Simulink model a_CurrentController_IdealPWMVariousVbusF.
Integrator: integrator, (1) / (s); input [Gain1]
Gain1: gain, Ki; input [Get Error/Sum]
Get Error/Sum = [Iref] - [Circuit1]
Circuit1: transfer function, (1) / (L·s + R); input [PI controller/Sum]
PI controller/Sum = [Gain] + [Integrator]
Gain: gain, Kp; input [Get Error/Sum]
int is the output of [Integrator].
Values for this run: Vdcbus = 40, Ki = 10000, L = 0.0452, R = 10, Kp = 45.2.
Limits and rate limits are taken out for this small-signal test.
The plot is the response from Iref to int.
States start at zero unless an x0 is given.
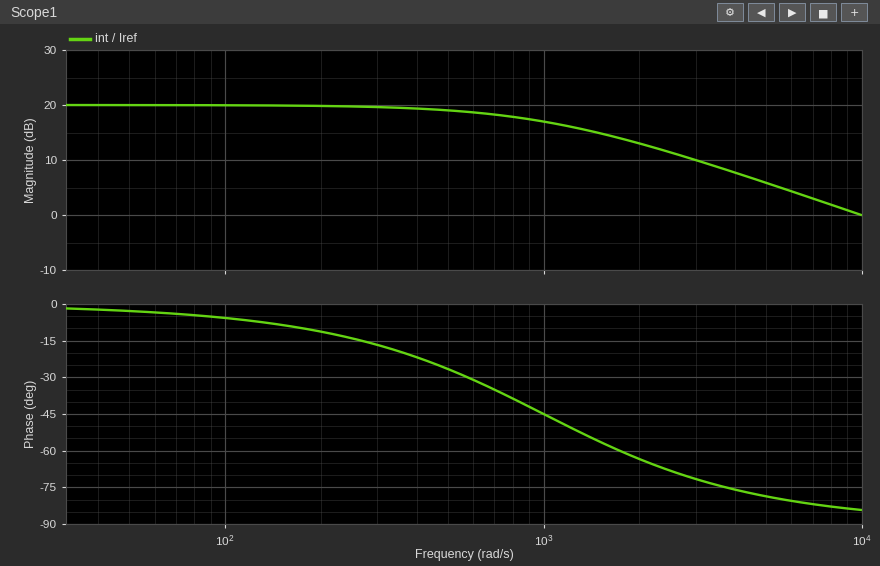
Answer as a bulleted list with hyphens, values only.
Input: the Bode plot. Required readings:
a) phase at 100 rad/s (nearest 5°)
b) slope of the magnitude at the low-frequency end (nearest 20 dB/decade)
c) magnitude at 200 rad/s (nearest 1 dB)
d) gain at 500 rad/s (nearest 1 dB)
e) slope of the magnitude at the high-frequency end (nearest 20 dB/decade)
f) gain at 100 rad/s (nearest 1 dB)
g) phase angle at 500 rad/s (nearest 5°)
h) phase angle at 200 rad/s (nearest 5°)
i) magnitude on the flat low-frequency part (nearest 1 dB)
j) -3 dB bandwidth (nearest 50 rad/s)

- -5°
- 0 dB/decade
- 20 dB
- 19 dB
- -20 dB/decade
- 20 dB
- -25°
- -10°
- 20 dB
- 1000 rad/s
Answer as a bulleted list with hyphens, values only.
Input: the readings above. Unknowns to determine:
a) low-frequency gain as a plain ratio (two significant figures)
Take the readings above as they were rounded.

- 10
